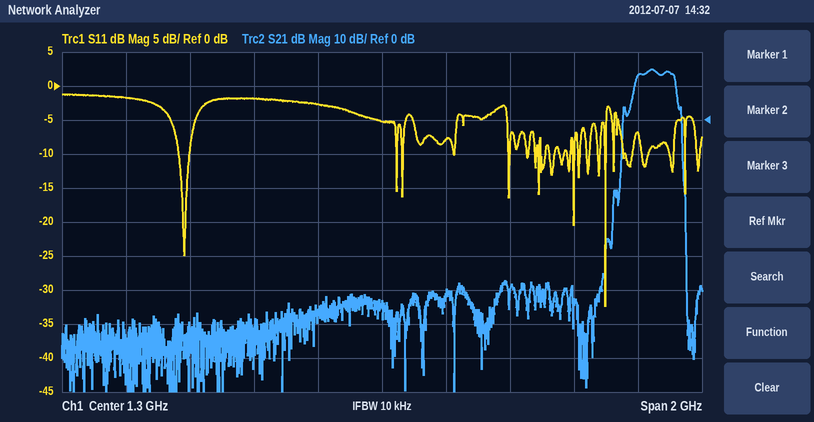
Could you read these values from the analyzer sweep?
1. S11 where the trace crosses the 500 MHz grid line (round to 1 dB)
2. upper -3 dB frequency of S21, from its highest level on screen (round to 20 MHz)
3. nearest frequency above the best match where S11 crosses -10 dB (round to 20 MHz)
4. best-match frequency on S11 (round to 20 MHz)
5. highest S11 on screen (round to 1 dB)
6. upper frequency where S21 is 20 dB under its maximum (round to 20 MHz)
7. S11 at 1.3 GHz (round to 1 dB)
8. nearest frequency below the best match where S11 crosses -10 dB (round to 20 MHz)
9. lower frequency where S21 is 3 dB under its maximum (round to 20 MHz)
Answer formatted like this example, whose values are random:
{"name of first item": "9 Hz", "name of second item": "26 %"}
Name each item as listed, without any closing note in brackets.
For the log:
{"S11 where the trace crosses the 500 MHz grid line": "-2 dB", "upper -3 dB frequency of S21, from its highest level on screen": "2.22 GHz", "nearest frequency above the best match where S11 crosses -10 dB": "2.00 GHz", "best-match frequency on S11": "2.00 GHz", "highest S11 on screen": "-1 dB", "upper frequency where S21 is 20 dB under its maximum": "2.24 GHz", "S11 at 1.3 GHz": "-5 dB", "nearest frequency below the best match where S11 crosses -10 dB": "2.00 GHz", "lower frequency where S21 is 3 dB under its maximum": "2.10 GHz"}
